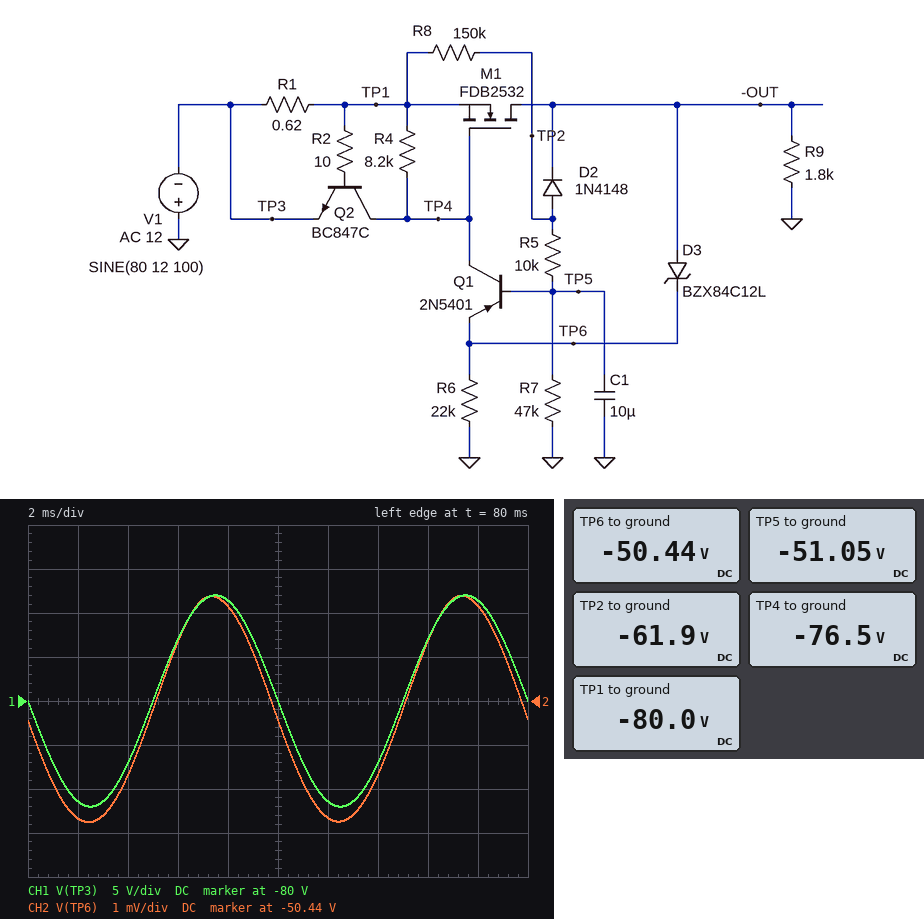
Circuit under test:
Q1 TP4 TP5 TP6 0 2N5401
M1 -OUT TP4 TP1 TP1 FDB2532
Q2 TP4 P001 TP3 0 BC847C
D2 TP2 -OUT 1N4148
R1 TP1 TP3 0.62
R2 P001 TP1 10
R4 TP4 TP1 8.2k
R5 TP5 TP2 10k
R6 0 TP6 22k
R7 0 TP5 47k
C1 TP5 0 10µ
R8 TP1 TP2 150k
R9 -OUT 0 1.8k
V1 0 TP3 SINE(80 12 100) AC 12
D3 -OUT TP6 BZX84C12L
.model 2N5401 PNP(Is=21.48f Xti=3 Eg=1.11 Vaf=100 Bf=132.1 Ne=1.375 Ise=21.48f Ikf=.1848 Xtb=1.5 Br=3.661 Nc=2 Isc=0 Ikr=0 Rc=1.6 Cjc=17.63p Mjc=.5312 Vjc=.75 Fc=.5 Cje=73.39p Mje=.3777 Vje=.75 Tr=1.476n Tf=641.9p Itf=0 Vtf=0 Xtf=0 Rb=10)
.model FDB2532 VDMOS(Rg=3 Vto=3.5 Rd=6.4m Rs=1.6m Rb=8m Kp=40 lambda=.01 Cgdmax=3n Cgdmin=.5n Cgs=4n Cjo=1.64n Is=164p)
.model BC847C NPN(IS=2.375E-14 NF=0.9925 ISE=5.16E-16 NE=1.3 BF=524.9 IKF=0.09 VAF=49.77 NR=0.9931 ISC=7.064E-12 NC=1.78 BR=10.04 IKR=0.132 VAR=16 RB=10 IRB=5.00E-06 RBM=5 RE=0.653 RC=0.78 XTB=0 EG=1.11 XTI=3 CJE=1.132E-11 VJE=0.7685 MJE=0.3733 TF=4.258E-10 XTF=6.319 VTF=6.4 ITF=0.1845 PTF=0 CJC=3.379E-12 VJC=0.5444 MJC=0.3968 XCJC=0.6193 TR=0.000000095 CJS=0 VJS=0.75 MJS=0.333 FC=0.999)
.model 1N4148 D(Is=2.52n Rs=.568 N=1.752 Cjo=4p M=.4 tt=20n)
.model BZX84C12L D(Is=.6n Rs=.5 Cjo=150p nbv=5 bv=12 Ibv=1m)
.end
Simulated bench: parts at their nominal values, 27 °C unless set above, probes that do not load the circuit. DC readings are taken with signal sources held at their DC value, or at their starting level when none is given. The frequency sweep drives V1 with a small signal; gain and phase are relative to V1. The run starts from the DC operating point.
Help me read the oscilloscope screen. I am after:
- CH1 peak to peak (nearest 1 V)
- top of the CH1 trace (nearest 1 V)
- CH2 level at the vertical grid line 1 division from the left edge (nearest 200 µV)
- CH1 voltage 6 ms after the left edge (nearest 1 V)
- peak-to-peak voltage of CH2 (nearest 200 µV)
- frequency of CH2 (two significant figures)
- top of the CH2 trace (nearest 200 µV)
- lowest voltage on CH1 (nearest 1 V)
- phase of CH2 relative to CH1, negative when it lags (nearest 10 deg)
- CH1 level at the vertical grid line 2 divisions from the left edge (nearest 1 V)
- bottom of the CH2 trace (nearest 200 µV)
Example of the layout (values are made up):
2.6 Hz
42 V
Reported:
24 V
-68 V
-50.4416 V
-73 V
5.2 mV
100 Hz
-50.4366 V
-92 V
0 deg
-87 V
-50.4418 V
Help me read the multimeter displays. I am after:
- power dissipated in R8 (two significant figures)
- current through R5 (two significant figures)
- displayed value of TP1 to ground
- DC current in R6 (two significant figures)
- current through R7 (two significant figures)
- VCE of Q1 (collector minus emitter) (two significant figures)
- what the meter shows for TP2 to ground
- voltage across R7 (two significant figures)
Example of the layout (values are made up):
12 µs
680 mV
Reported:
2.2 mW
1.1 mA
-80.0 V
2.3 mA
1.1 mA
-26 V
-61.9 V
51 V
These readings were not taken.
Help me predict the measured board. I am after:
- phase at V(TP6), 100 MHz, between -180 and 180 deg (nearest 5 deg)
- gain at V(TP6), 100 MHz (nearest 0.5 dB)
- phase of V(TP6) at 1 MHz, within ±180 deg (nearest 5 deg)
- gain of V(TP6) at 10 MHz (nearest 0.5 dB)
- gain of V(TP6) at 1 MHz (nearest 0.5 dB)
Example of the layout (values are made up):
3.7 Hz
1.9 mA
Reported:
-165 deg
-10.0 dB
-115 deg
-6.5 dB
-13.5 dB
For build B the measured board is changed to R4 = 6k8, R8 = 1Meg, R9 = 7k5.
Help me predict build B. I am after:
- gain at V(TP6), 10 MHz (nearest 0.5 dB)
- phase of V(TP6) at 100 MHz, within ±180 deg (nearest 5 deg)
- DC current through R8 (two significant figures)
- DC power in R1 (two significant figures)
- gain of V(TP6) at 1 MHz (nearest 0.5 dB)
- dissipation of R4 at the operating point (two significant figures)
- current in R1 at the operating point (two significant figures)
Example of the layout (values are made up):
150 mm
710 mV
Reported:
-8.0 dB
-160 deg
18 µA
85 µW
-15.0 dB
1.7 mW
12 mA
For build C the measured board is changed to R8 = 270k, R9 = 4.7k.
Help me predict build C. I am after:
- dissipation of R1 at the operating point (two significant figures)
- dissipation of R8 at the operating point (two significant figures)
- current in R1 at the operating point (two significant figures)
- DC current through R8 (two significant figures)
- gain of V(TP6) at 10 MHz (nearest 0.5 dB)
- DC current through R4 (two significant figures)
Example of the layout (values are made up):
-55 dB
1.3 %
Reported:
170 µW
1.2 mW
17 mA
67 µA
-7.0 dB
410 µA
